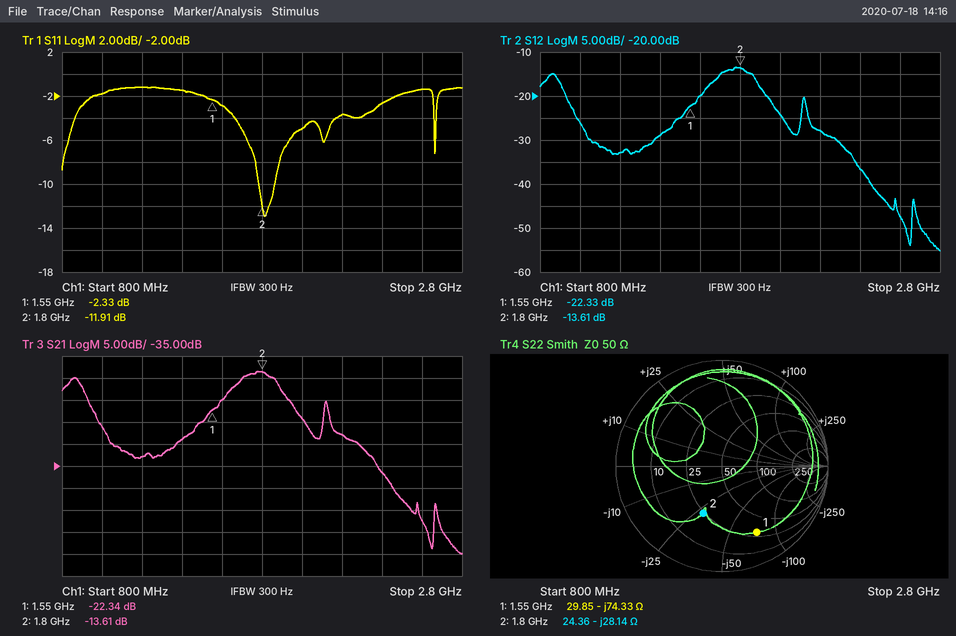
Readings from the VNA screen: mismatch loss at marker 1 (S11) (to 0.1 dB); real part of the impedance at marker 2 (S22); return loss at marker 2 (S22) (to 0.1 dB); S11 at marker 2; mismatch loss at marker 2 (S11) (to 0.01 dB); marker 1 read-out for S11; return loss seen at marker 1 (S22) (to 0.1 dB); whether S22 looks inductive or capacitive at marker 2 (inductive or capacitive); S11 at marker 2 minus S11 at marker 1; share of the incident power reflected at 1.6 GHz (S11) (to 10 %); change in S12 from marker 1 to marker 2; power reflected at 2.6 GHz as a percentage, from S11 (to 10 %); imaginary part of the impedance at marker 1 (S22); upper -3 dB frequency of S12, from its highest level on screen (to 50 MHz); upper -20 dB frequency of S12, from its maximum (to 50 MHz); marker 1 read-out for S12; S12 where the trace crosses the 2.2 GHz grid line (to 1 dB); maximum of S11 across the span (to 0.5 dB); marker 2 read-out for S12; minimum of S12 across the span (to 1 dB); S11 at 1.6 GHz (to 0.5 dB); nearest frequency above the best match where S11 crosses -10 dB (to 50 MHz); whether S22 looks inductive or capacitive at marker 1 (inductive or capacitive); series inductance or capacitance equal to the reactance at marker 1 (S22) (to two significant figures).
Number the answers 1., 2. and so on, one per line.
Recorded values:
1. 3.8 dB
2. 24.36 Ω
3. 6.4 dB
4. -11.91 dB
5. 0.29 dB
6. -2.33 dB
7. 3.0 dB
8. capacitive
9. -9.58 dB
10. 50 %
11. 8.72 dB
12. 70 %
13. -74.33 Ω
14. 1.90 GHz
15. 2.35 GHz
16. -22.33 dB
17. -28 dB
18. -1.0 dB
19. -13.61 dB
20. -55 dB
21. -3.0 dB
22. 1.85 GHz
23. capacitive
24. 1.4 pF
